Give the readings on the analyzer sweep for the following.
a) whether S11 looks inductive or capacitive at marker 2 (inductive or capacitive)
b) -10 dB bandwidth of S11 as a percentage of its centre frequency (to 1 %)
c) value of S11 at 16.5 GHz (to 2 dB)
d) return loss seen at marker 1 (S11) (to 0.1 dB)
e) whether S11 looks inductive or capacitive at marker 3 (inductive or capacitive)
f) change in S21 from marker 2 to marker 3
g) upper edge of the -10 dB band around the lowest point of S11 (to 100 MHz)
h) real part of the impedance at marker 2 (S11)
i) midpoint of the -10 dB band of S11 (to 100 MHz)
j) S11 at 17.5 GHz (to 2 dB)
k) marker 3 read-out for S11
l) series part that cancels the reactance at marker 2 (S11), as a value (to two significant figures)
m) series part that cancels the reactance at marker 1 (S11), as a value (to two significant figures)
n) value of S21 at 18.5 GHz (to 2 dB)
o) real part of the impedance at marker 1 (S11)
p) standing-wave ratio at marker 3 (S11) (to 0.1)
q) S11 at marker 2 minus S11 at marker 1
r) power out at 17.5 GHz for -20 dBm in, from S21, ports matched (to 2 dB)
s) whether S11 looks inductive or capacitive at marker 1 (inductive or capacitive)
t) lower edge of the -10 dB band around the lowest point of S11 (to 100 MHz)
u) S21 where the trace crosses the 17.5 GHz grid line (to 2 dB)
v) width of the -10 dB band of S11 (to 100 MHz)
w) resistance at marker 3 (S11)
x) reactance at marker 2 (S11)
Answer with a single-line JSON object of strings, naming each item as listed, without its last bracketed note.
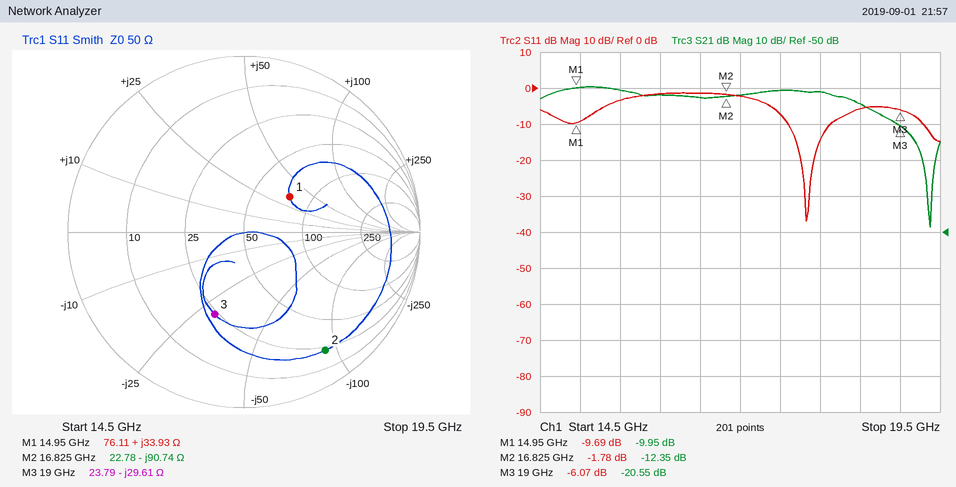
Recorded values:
{"whether S11 looks inductive or capacitive at marker 2": "capacitive", "-10 dB bandwidth of S11 as a percentage of its centre frequency": "3 %", "value of S11 at 16.5 GHz": "-2 dB", "return loss seen at marker 1 (S11)": "9.7 dB", "whether S11 looks inductive or capacitive at marker 3": "capacitive", "change in S21 from marker 2 to marker 3": "-8.20 dB", "upper edge of the -10 dB band around the lowest point of S11": "18.1 GHz", "real part of the impedance at marker 2": "22.78 Ω", "midpoint of the -10 dB band of S11": "17.9 GHz", "S11 at 17.5 GHz": "-8 dB", "marker 3 read-out for S11": "-6.07 dB", "series part that cancels the reactance at marker 2 (S11), as a value": "860 pH", "series part that cancels the reactance at marker 1 (S11), as a value": "310 fF", "value of S21 at 18.5 GHz": "-14 dB", "real part of the impedance at marker 1": "76.11 Ω", "standing-wave ratio at marker 3 (S11)": "3.0", "S11 at marker 2 minus S11 at marker 1": "7.91 dB", "power out at 17.5 GHz for -20 dBm in, from S21, ports matched": "-30 dBm", "whether S11 looks inductive or capacitive at marker 1": "inductive", "lower edge of the -10 dB band around the lowest point of S11": "17.6 GHz", "S21 where the trace crosses the 17.5 GHz grid line": "-10 dB", "width of the -10 dB band of S11": "500 MHz", "resistance at marker 3": "23.79 Ω", "reactance at marker 2": "-90.74 Ω"}
